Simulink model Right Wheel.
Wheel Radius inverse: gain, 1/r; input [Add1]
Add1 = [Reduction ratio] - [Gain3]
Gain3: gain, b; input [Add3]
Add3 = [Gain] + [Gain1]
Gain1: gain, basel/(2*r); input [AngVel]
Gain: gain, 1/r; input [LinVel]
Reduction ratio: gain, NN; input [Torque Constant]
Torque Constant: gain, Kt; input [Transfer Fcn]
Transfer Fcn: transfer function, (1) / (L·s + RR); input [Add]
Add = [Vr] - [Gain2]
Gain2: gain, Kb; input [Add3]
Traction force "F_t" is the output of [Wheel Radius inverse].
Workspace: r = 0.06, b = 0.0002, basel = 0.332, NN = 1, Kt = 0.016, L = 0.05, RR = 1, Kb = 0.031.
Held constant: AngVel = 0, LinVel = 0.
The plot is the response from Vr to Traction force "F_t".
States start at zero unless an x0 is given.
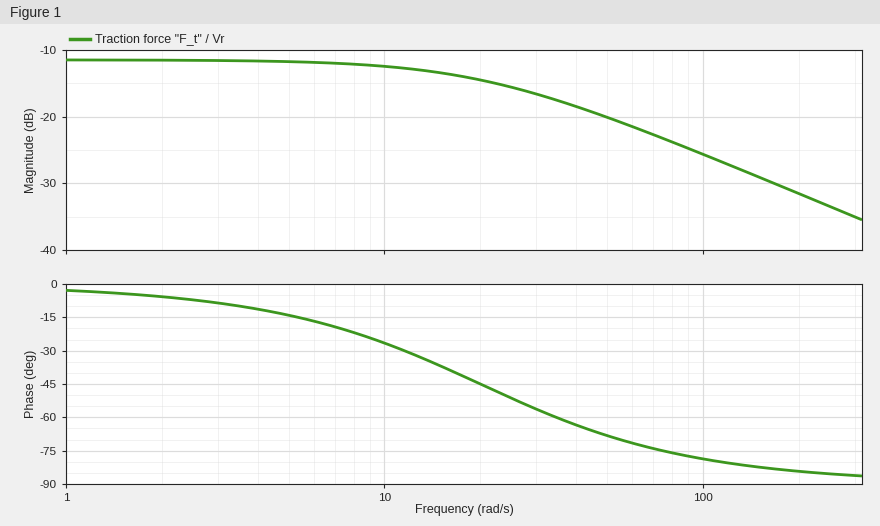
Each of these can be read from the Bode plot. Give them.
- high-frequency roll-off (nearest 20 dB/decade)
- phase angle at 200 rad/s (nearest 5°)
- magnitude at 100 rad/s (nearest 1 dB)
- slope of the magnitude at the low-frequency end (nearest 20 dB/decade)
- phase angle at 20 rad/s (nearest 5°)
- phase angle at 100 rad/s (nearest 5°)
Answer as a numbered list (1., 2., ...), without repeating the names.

1. -20 dB/decade
2. -85°
3. -26 dB
4. 0 dB/decade
5. -45°
6. -80°
